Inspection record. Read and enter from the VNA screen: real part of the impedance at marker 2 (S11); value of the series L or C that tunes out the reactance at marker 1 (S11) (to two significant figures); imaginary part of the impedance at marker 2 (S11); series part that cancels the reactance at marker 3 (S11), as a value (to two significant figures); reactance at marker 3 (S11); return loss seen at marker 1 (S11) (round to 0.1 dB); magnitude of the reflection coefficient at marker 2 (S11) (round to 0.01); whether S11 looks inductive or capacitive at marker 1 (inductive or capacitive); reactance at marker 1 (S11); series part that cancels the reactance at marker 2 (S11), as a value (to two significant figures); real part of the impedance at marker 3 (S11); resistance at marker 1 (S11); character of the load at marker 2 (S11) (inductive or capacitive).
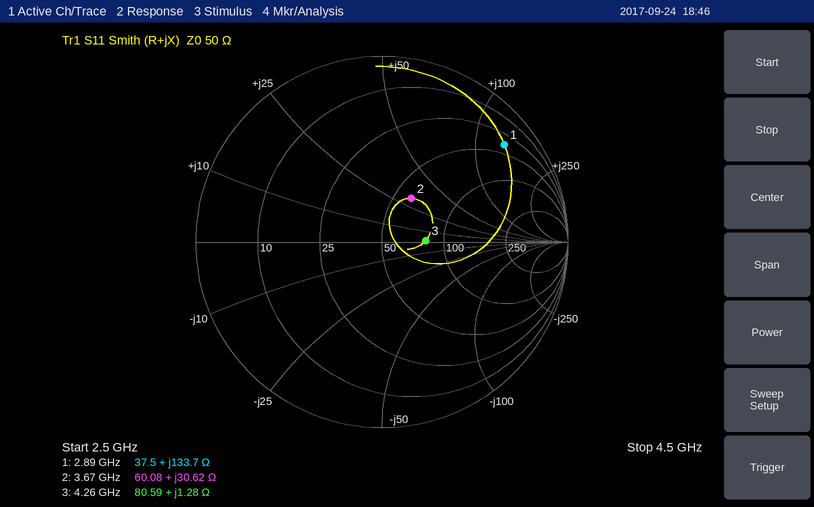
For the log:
60.08 Ω
410 fF
+30.62 Ω
29 pF
+1.28 Ω
1.5 dB
0.28
inductive
+133.7 Ω
1.4 pF
80.59 Ω
37.5 Ω
inductive
